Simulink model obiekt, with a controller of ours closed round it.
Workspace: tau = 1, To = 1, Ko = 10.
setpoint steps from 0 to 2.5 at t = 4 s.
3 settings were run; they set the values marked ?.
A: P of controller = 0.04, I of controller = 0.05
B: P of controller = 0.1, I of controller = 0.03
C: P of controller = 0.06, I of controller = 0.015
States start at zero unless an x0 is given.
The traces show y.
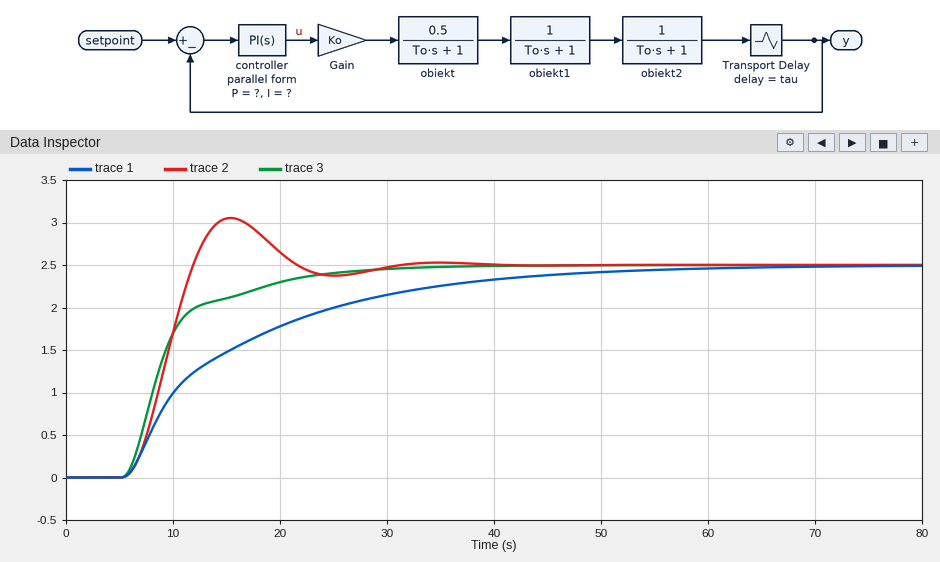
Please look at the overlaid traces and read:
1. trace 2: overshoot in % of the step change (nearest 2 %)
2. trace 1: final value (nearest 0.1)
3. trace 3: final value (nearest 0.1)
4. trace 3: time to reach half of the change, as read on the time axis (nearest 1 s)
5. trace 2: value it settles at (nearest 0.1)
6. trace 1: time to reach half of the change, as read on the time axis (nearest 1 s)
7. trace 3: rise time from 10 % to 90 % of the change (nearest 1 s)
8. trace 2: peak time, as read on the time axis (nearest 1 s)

22 %
2.5
2.5
9 s
2.5
12 s
12 s
15 s
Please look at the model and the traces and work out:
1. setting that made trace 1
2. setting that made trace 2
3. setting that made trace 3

C
A
B
